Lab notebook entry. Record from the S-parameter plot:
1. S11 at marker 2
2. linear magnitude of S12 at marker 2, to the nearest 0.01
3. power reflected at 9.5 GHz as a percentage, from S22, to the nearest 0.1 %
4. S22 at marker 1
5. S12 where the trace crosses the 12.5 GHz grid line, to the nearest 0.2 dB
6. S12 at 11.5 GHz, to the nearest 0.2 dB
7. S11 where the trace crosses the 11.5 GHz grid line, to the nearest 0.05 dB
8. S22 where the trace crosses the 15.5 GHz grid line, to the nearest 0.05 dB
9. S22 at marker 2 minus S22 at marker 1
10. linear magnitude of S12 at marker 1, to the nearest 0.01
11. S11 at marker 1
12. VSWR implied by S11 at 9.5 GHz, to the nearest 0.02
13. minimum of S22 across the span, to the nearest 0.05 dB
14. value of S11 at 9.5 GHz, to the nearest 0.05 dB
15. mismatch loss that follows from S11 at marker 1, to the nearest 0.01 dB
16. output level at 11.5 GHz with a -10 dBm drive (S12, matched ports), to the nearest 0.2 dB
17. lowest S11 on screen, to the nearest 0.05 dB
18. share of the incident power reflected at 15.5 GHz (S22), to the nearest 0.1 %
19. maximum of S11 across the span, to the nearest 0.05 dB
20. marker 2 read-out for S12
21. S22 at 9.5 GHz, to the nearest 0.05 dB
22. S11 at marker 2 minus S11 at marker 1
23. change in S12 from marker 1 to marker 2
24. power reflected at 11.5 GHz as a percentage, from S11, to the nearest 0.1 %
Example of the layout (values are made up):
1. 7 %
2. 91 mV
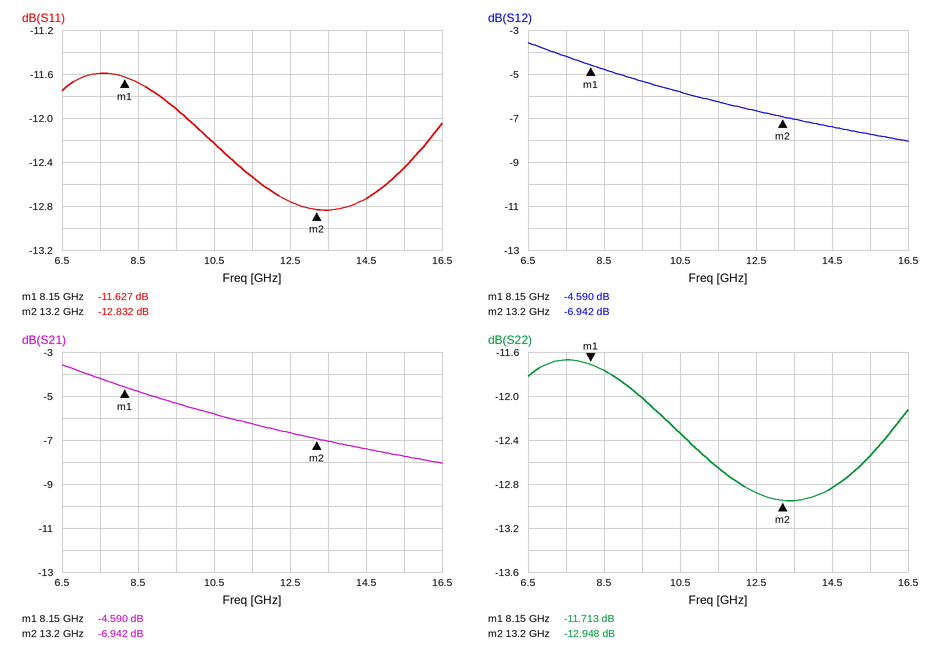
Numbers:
1. -12.832 dB
2. 0.45
3. 6.3 %
4. -11.713 dB
5. -6.6 dB
6. -6.2 dB
7. -12.55 dB
8. -12.55 dB
9. -1.235 dB
10. 0.59
11. -11.627 dB
12. 1.68
13. -12.95 dB
14. -11.90 dB
15. 0.31 dB
16. -16.2 dBm
17. -12.85 dB
18. 5.6 %
19. -11.60 dB
20. -6.942 dB
21. -12.00 dB
22. -1.205 dB
23. -2.352 dB
24. 5.6 %
